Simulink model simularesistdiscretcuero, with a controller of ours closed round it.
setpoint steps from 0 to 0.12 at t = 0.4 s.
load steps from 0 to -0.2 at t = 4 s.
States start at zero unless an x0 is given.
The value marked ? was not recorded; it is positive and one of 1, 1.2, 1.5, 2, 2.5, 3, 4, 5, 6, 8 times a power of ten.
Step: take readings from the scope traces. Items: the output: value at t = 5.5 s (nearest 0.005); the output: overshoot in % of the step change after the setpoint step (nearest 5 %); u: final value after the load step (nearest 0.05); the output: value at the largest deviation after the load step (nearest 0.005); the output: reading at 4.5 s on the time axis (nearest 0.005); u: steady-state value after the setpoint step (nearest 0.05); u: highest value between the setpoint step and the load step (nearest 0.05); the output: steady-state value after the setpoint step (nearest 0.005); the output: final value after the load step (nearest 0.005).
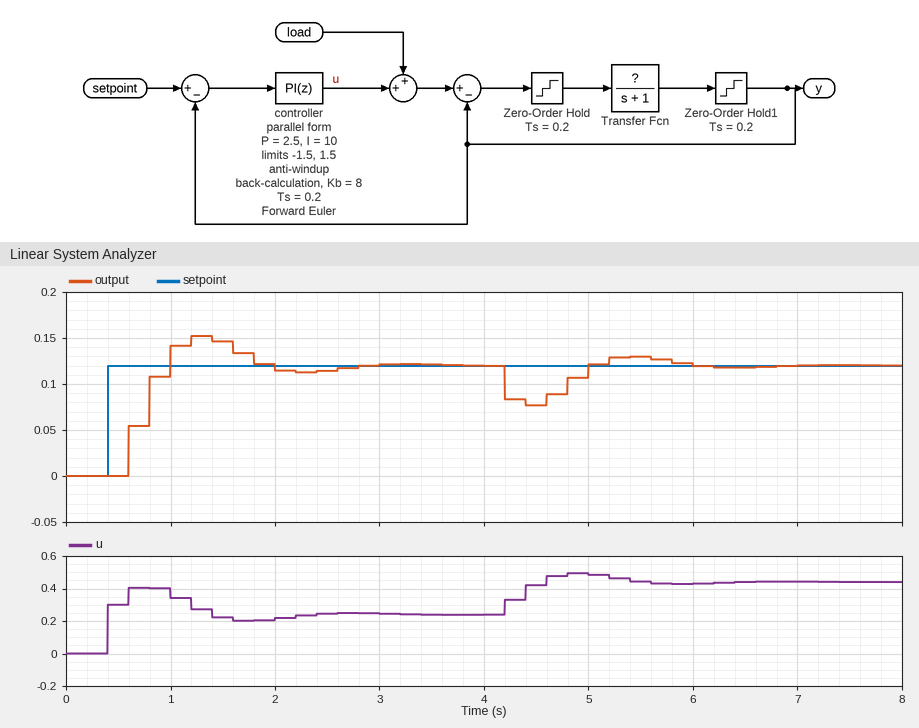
0.130
25 %
0.45
0.075
0.075
0.25
0.40
0.120
0.120
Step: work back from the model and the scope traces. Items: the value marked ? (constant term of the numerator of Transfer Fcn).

1
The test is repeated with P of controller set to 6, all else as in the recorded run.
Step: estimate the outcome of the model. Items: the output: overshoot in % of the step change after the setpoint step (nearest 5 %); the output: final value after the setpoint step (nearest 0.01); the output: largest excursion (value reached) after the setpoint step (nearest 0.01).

10 %
0.12
0.13
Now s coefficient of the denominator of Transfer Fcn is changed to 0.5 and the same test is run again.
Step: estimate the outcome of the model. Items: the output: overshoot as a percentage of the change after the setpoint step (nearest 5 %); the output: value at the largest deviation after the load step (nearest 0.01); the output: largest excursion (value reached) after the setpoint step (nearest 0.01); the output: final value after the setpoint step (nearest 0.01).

10 %
0.05
0.13
0.12
